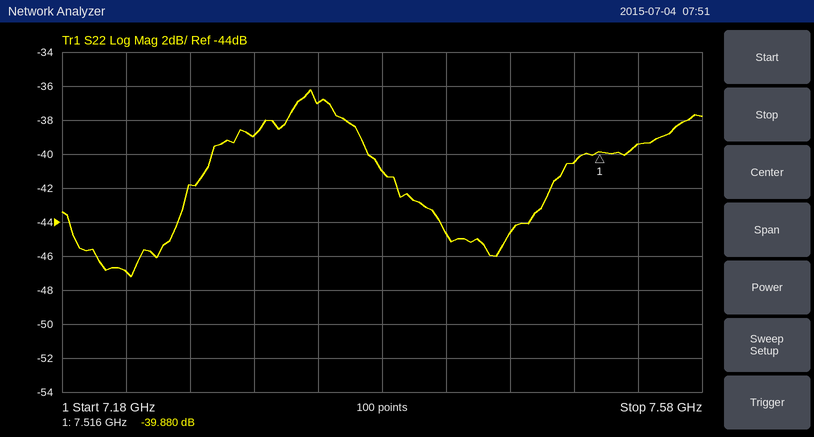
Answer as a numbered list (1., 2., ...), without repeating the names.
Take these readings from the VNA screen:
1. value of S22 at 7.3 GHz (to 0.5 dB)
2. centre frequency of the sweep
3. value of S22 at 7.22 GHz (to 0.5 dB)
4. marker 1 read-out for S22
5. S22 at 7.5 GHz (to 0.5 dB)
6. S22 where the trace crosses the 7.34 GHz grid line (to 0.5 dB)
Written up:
1. -39.0 dB
2. 7.38 GHz
3. -47.0 dB
4. -39.880 dB
5. -40.5 dB
6. -37.0 dB
